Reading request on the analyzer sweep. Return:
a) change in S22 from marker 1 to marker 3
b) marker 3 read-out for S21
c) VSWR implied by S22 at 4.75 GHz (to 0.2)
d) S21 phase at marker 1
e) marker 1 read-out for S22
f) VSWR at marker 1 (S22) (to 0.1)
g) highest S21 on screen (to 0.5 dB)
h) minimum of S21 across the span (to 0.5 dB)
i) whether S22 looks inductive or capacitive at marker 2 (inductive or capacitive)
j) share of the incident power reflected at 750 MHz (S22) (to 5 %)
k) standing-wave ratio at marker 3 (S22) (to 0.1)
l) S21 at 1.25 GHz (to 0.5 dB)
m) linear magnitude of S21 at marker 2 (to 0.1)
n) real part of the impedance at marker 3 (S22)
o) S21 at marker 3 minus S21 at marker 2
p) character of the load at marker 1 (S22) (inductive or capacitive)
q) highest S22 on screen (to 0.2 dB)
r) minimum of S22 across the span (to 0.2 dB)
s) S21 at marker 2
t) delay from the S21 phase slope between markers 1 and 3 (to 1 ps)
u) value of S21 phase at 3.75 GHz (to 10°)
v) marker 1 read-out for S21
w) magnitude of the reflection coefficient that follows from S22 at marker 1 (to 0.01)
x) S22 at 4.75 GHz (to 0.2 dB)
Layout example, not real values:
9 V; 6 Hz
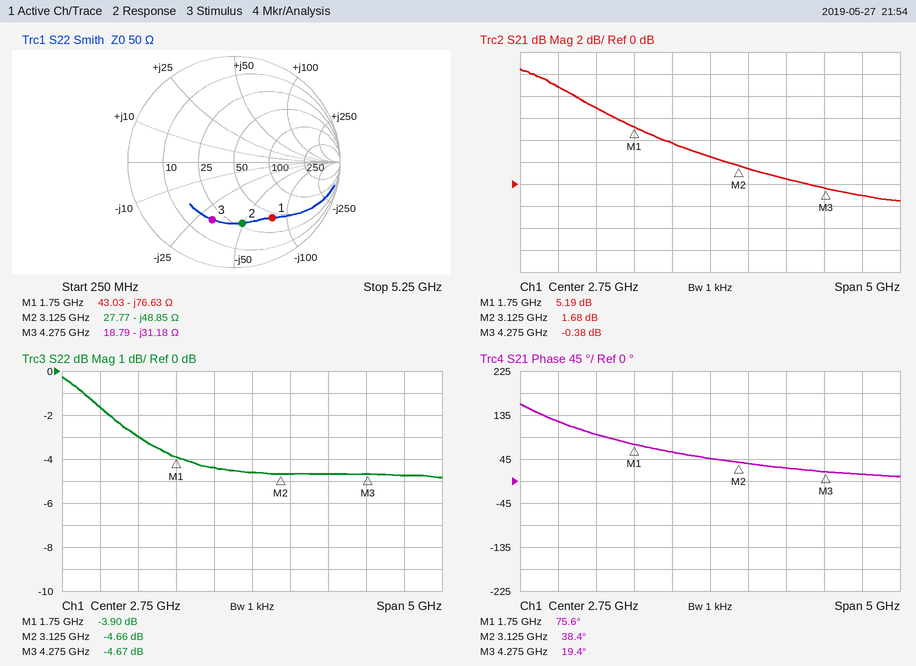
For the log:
-0.77 dB; -0.38 dB; 3.8; 75.6°; -3.90 dB; 4.5; 10.5 dB; -1.5 dB; capacitive; 70 %; 3.8; 7.0 dB; 1.2; 18.79 Ω; -2.06 dB; capacitive; -0.2 dB; -4.8 dB; 1.68 dB; 62 ps; 30°; 5.19 dB; 0.64; -4.8 dB
